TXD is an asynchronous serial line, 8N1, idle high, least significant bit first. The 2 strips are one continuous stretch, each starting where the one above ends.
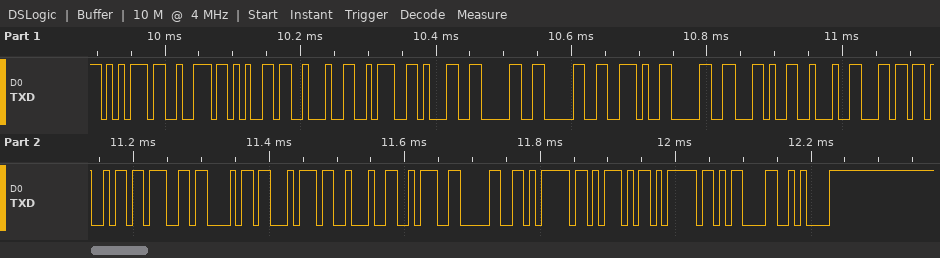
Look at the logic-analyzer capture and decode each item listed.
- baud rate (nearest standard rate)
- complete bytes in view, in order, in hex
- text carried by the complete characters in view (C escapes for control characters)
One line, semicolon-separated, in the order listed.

115200 baud; 75 72 65 22 3A 31 30 30 2E 30 2C 22 6C 69 67 68 74 22 3A 30 7D 5D 7D 0D 0A; "ure\":100.0,\"light\":0}]}\r\n"
